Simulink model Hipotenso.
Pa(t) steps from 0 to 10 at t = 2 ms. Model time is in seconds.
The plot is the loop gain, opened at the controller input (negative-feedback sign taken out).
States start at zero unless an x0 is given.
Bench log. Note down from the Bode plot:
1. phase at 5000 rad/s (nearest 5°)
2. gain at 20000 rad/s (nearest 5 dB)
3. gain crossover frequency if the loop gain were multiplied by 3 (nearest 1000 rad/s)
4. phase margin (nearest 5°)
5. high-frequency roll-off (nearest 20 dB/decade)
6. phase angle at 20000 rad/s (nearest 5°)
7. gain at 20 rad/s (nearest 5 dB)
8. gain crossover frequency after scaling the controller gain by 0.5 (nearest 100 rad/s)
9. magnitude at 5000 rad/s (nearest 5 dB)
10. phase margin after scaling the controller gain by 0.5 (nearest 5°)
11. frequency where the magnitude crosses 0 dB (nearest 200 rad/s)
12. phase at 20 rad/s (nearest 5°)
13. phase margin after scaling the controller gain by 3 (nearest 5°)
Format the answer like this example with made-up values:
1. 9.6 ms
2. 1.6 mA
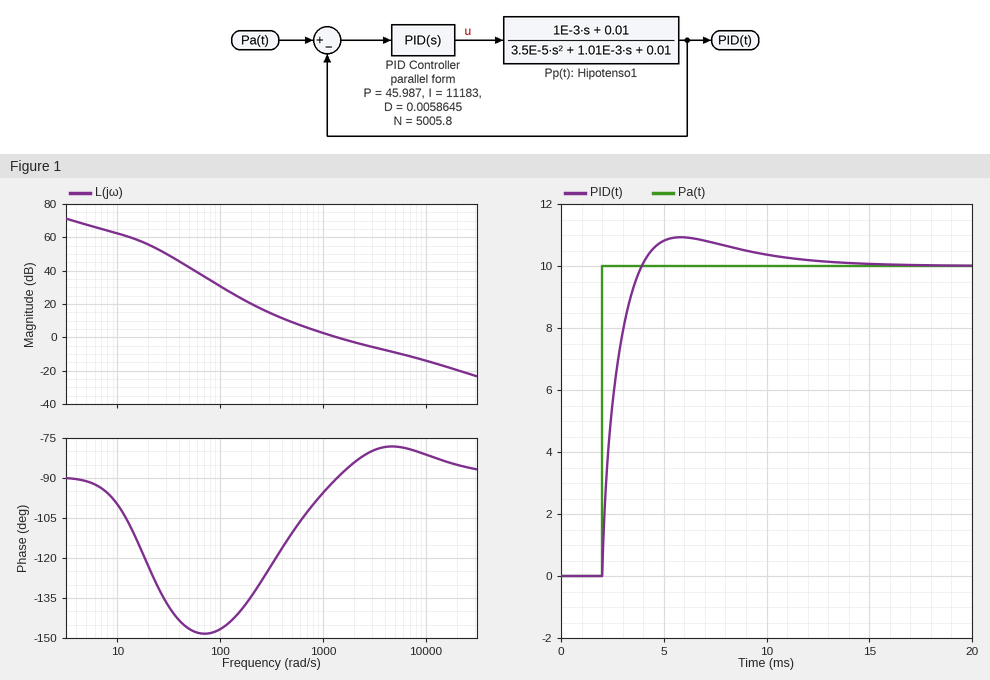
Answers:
1. -80°
2. -20 dB
3. 5000 rad/s
4. 90°
5. -20 dB/decade
6. -85°
7. 55 dB
8. 700 rad/s
9. -10 dB
10. 75°
11. 1400 rad/s
12. -125°
13. 100°
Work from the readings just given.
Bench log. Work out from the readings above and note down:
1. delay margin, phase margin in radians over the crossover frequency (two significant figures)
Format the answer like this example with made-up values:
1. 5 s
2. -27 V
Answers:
1. 0.0011 s
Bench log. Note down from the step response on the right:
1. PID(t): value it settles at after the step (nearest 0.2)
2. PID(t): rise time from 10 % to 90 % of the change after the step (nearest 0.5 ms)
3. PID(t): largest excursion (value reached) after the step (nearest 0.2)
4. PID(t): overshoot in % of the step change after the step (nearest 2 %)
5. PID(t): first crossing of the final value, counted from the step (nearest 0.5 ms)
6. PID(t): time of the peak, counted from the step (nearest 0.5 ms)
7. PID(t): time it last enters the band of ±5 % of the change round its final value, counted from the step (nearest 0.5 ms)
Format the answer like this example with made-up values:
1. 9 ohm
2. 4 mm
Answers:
1. 10.0
2. 1.5 ms
3. 11.0
4. 10 %
5. 2.0 ms
6. 4.0 ms
7. 7.0 ms
